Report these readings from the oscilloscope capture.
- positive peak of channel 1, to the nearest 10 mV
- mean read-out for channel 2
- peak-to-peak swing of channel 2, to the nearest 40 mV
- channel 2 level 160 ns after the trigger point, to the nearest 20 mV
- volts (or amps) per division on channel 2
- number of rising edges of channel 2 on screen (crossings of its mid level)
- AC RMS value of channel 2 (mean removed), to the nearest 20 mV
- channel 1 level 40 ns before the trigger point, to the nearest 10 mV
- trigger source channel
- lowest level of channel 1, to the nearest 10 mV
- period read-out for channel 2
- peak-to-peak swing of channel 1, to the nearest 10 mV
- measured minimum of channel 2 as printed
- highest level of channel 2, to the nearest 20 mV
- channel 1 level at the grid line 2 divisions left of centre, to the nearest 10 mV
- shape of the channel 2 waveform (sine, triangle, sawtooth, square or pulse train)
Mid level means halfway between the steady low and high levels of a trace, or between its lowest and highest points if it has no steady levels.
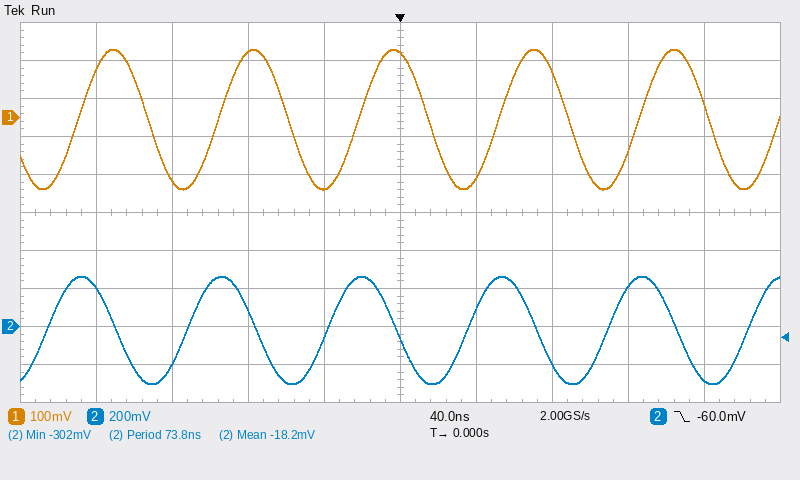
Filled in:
180 mV
-18.2 mV
560 mV
-280 mV
200 mV
6
200 mV
-190 mV
channel 2
-190 mV
73.8 ns
370 mV
-302 mV
260 mV
170 mV
sine
